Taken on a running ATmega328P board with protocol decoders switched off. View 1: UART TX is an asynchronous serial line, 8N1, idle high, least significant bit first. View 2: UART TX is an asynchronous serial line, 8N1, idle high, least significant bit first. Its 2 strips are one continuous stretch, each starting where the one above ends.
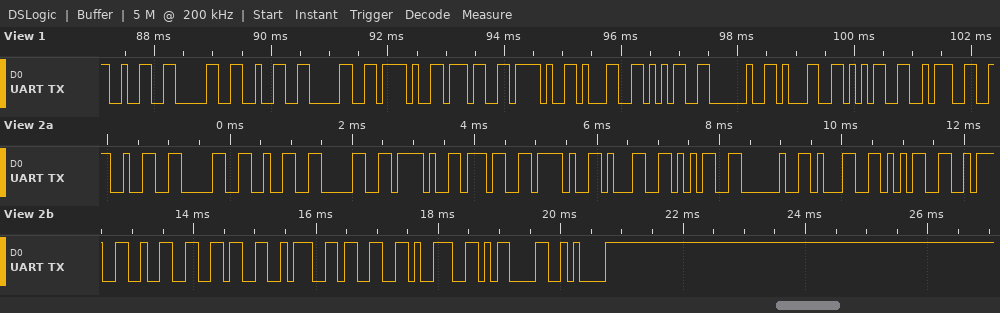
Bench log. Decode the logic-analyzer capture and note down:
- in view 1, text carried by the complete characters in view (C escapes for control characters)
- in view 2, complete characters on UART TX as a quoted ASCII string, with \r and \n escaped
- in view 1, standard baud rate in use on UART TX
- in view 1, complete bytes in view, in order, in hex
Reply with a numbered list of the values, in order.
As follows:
1. "2020/7/15 15:"
2. "2020/7/15 15:26:39\r\n"
3. 9600 baud
4. 32 30 32 30 2F 37 2F 31 35 20 31 35 3A
